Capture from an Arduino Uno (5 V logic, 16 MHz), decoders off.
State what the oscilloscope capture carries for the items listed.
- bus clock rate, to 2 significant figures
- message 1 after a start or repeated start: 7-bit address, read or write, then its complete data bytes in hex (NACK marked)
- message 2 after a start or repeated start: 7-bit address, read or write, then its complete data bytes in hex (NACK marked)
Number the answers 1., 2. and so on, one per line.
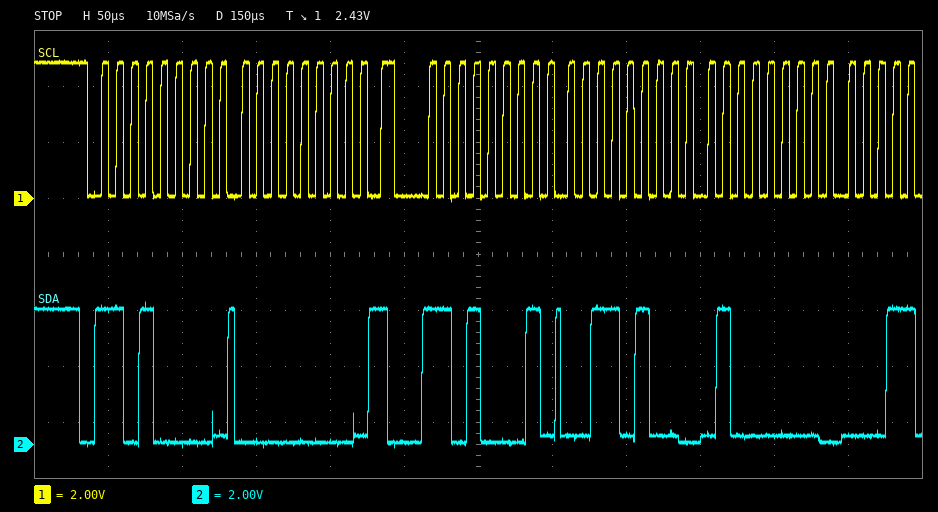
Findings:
1. 100 kHz
2. 0x68 write: 00
3. 0x68 read: 34 40
